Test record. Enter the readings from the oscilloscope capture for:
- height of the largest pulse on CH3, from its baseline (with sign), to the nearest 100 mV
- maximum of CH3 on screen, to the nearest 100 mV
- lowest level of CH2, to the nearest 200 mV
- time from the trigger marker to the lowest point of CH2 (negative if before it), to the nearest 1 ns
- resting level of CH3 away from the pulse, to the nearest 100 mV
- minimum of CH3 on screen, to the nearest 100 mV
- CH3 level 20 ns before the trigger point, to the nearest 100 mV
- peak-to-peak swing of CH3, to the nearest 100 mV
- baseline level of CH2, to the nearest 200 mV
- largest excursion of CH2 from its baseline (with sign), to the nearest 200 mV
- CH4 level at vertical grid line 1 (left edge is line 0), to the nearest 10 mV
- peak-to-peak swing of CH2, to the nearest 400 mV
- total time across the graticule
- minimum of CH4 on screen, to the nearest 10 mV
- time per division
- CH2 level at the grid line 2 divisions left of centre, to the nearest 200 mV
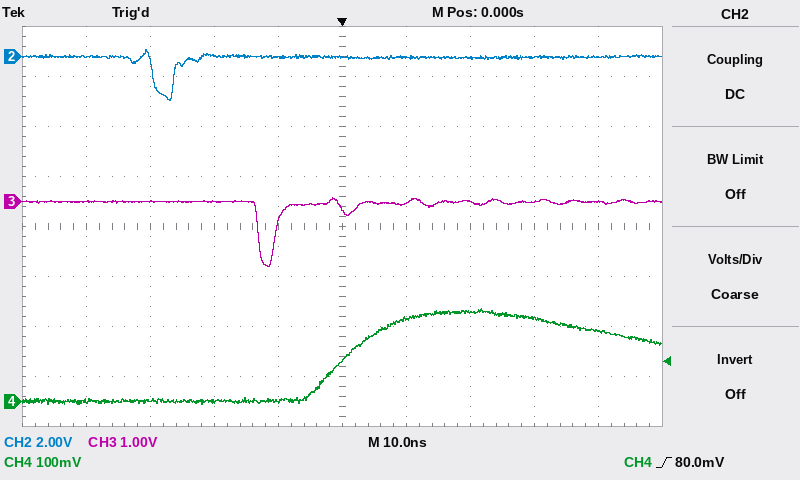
-1.3 V
100 mV
-1.8 V
-27 ns
0.0 V
-1.3 V
0.0 V
1.4 V
0.0 V
-1.8 V
0 mV
2.0 V
100 ns
-10 mV
10 ns
0.0 V
